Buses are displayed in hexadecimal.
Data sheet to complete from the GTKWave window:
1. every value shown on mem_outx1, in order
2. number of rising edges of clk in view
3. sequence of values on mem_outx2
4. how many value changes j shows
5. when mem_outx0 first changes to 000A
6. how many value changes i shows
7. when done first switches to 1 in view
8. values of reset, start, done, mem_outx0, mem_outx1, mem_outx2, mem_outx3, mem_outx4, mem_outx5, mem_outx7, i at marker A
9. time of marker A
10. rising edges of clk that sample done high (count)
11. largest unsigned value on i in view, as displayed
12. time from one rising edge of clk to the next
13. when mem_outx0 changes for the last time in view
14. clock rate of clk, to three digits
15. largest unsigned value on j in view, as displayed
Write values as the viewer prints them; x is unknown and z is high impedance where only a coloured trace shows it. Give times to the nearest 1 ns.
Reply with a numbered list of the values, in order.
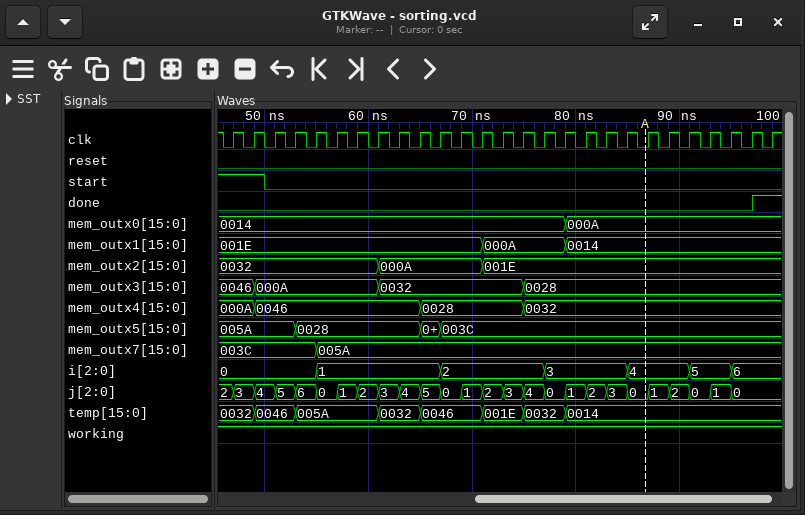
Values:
1. 001E, 000A, 0014
2. 27
3. 0032, 000A, 001E
4. 25
5. 79 ns
6. 6
7. 97 ns
8. reset=0, start=0, done=0, mem_outx0=000A, mem_outx1=0014, mem_outx2=001E, mem_outx3=0028, mem_outx4=0032, mem_outx5=003C, mem_outx7=005A, i=4
9. 87 ns
10. 1
11. 6
12. 2 ns
13. 79 ns
14. 500 MHz
15. 6
